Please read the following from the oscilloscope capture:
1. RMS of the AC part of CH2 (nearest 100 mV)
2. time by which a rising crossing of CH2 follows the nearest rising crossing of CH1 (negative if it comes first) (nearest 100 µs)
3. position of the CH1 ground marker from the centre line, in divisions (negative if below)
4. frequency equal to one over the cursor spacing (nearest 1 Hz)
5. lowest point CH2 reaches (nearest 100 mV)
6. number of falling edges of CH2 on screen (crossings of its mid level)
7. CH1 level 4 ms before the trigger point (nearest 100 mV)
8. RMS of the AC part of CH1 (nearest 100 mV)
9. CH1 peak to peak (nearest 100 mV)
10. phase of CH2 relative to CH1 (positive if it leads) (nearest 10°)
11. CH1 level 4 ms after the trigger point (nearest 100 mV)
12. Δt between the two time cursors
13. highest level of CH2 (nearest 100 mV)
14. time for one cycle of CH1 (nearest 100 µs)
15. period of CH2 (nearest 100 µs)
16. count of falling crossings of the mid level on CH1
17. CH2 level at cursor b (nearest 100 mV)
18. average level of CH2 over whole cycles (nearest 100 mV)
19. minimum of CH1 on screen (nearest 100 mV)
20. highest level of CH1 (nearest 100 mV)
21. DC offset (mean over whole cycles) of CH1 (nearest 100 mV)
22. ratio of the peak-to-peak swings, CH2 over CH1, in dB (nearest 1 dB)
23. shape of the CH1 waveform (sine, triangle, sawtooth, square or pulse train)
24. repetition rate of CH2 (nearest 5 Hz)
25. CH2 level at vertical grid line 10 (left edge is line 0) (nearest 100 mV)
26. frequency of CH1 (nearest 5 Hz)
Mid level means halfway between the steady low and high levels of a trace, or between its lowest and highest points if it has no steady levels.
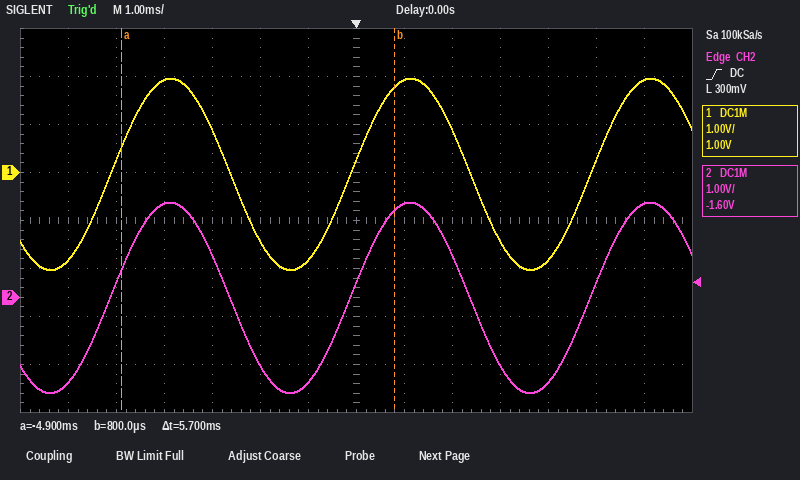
1.4 V
0.0 ms
+1.0 div
175 Hz
-2.0 V
2
1.9 V
1.4 V
4.0 V
0°
-1.8 V
5.7 ms
2.0 V
5.0 ms
5.0 ms
2
1.8 V
0.0 V
-2.0 V
2.0 V
0.0 V
0 dB
sine
200 Hz
-1.4 V
200 Hz
